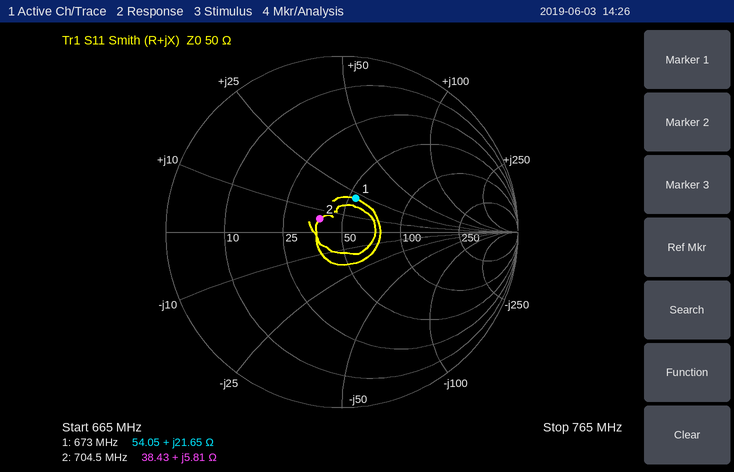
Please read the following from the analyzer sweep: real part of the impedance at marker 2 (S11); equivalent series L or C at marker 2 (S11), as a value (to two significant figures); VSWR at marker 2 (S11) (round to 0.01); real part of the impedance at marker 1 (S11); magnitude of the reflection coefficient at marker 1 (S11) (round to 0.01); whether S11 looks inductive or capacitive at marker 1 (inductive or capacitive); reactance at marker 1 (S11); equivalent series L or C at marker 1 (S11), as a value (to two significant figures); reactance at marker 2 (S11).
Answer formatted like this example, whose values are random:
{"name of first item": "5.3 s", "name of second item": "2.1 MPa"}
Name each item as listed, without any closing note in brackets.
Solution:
{"real part of the impedance at marker 2": "38.43 Ω", "equivalent series L or C at marker 2 (S11), as a value": "1.3 nH", "VSWR at marker 2 (S11)": "1.34", "real part of the impedance at marker 1": "54.05 Ω", "magnitude of the reflection coefficient at marker 1 (S11)": "0.21", "whether S11 looks inductive or capacitive at marker 1": "inductive", "reactance at marker 1": "+21.65 Ω", "equivalent series L or C at marker 1 (S11), as a value": "5.1 nH", "reactance at marker 2": "+5.81 Ω"}
